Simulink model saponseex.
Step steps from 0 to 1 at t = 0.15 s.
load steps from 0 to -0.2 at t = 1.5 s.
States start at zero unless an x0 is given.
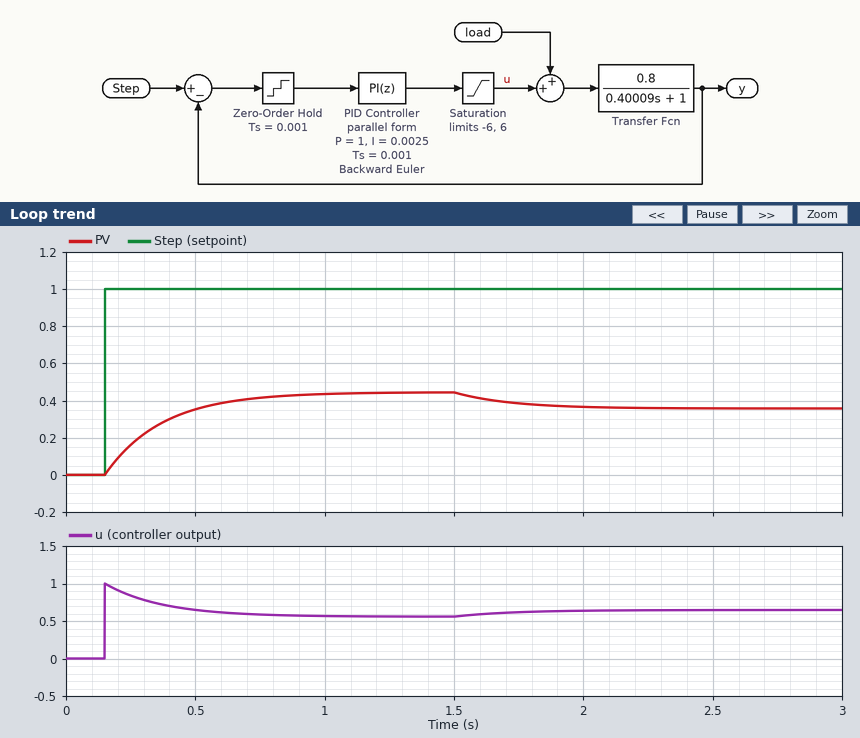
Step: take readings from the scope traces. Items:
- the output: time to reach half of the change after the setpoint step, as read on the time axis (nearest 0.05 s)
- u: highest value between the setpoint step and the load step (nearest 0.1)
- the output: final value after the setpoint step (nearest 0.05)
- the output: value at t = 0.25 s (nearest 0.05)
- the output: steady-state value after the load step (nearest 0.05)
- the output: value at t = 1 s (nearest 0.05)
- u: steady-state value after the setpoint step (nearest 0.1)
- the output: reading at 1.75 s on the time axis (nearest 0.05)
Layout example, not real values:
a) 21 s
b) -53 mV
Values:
a) 0.30 s
b) 1.0
c) 0.45
d) 0.15
e) 0.35
f) 0.45
g) 0.6
h) 0.40
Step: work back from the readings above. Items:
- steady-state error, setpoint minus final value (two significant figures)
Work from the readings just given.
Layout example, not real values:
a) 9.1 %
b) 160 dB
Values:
a) 0.55
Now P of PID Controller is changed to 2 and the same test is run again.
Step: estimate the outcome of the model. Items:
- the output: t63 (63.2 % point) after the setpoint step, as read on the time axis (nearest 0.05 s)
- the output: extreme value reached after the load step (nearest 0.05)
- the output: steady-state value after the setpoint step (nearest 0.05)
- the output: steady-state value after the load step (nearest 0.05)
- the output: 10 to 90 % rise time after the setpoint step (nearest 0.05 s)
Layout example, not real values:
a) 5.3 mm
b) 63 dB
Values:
a) 0.30 s
b) 0.55
c) 0.60
d) 0.55
e) 0.35 s
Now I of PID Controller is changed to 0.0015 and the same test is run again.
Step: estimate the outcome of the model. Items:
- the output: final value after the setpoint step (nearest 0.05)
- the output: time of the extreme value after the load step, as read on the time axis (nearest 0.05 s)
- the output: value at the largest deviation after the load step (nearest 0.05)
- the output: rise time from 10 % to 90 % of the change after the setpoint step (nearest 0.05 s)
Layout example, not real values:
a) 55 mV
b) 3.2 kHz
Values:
a) 0.45
b) 3.00 s
c) 0.35
d) 0.50 s
